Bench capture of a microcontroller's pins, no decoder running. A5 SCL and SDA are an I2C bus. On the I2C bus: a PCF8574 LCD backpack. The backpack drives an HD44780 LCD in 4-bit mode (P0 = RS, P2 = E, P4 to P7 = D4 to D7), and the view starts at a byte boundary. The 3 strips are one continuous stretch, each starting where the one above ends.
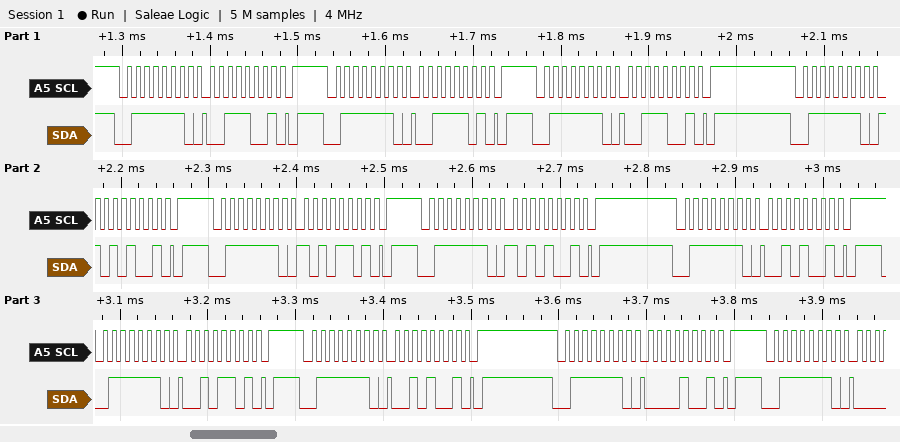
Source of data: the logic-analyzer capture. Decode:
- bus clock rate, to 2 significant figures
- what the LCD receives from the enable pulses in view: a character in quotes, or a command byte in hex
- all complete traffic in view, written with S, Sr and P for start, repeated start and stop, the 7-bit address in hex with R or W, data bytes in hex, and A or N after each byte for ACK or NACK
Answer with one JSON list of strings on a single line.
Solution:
["100 kHz", "':'", "S 3FW A 39 A P S 3FW A 3D A P S 3FW A 39 A P S 3FW A A9 A P S 3FW A AD A P S 3FW A A9 A P S 3FW A 29 A P S 3FW A 2D A P S 3FW A 29 A P S 3FW A 09 A P S 3FW A"]
